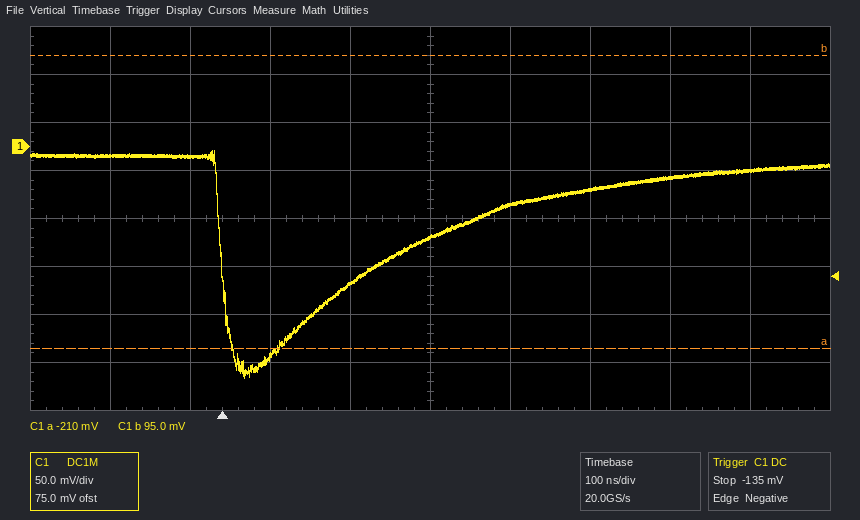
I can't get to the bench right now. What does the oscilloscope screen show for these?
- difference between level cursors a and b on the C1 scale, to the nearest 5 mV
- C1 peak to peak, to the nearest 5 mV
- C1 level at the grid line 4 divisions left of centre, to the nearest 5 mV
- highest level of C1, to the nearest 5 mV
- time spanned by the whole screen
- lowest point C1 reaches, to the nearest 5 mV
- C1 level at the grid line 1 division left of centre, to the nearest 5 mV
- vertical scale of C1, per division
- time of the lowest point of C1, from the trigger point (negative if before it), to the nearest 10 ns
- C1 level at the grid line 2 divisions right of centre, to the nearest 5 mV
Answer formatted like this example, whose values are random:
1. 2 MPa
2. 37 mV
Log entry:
1. 305 mV
2. 235 mV
3. -10 mV
4. -5 mV
5. 1 µs
6. -240 mV
7. -145 mV
8. 50 mV
9. +30 ns
10. -45 mV
